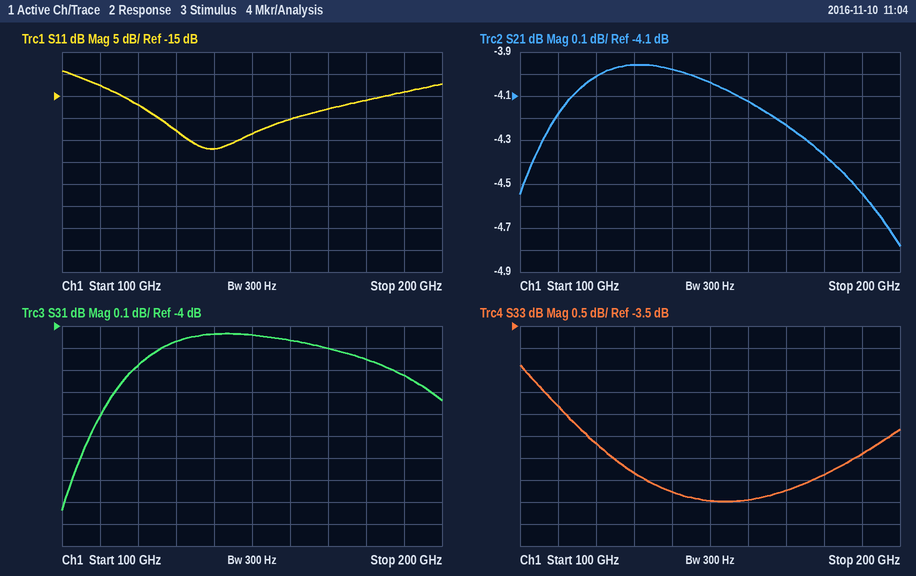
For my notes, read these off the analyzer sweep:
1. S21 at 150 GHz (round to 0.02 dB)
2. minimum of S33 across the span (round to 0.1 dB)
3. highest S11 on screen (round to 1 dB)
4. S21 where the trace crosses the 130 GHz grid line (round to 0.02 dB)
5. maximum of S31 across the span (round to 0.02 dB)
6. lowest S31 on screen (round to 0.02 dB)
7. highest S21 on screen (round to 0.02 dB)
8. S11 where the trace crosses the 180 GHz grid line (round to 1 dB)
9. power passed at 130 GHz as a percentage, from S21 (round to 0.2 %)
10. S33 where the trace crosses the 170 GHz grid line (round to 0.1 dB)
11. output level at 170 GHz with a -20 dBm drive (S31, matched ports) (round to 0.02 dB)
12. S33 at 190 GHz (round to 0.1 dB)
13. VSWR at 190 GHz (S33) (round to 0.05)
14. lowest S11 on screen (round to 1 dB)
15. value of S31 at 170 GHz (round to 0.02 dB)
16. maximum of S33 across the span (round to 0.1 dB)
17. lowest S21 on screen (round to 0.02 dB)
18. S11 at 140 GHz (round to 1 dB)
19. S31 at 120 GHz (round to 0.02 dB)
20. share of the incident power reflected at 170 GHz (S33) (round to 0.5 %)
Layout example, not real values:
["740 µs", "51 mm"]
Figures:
["-4.04 dB", "-7.5 dB", "-9 dB", "-3.96 dB", "-4.04 dB", "-4.84 dB", "-3.96 dB", "-16 dB", "40.2 %", "-7.2 dB", "-24.10 dBm", "-6.4 dB", "2.85", "-27 dB", "-4.10 dB", "-4.4 dB", "-4.78 dB", "-27 dB", "-4.18 dB", "19.0 %"]
